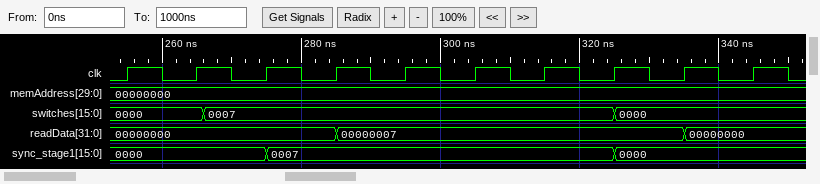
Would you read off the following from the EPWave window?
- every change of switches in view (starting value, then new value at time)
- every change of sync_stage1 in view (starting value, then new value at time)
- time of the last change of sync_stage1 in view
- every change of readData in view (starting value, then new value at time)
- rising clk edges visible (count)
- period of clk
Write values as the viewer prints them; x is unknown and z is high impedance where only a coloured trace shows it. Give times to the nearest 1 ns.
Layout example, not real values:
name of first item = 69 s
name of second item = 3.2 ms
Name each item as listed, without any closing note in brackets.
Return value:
every change of switches in view = 0000, 0007 at 266 ns, 0000 at 325 ns
every change of sync_stage1 in view = 0000, 0007 at 275 ns, 0000 at 325 ns
time of the last change of sync_stage1 in view = 325 ns
every change of readData in view = 00000000, 00000007 at 285 ns, 00000000 at 335 ns
rising clk edges visible = 10
period of clk = 10 ns
